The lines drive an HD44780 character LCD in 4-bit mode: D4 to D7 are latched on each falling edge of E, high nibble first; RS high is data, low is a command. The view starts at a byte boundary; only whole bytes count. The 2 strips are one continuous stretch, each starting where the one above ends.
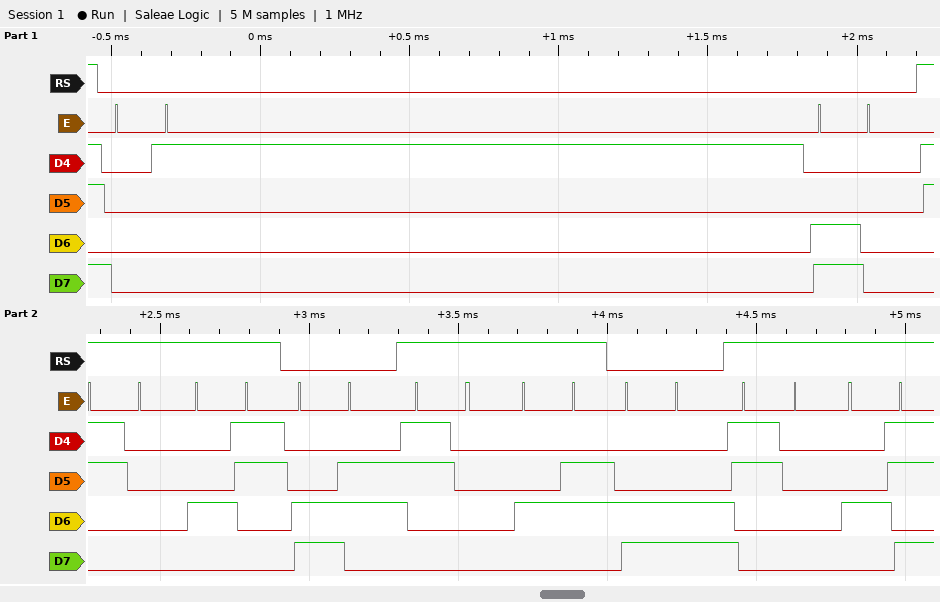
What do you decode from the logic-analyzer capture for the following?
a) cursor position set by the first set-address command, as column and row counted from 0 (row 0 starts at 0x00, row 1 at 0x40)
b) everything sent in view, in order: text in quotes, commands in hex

column 0, row 1
0x01 0xC0 "0C" 0xC6 "0F" 0xCC "0K"
